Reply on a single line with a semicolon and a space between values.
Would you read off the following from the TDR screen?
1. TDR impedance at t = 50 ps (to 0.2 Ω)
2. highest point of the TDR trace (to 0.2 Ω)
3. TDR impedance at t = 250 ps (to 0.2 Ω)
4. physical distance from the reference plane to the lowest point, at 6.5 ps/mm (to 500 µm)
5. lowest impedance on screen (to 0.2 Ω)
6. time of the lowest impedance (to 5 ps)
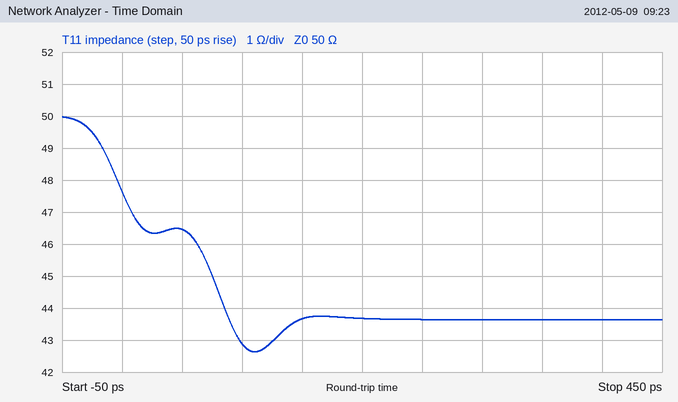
46.4 Ω; 50.0 Ω; 43.6 Ω; 8.5 mm; 42.6 Ω; 110 ps
